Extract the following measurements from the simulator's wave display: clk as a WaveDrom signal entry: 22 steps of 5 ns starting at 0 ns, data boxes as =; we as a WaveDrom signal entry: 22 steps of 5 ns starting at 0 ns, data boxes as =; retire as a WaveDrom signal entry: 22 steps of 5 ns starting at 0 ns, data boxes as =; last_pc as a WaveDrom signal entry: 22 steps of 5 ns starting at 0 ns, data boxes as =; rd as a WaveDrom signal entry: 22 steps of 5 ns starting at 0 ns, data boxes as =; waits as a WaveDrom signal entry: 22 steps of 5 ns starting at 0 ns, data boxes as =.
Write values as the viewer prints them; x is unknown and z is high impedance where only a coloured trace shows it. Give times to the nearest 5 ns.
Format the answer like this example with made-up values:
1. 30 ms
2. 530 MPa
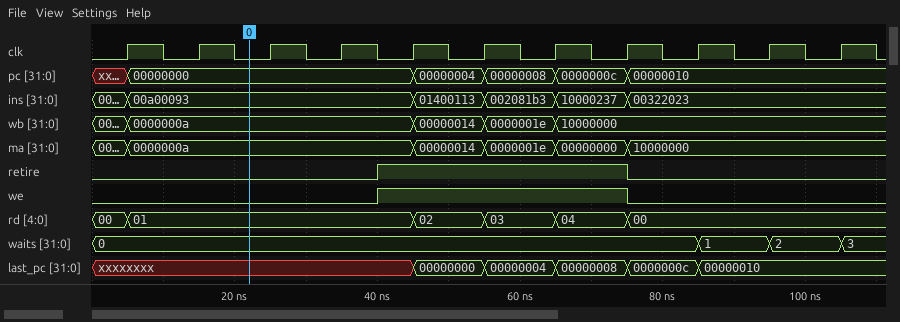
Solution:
1. {name: 'clk', wave: '0101010101010101010101'}
2. {name: 'we', wave: '0.......1......0......'}
3. {name: 'retire', wave: '0.......1......0......'}
4. {name: 'last_pc', wave: 'x........=.=.=.=.=....', data: '00000000 00000004 00000008 0000000c 00000010'}
5. {name: 'rd', wave: '==.......=.=.=.=......', data: '00 01 02 03 04 00'}
6. {name: 'waits', wave: '=................=.=.=', data: '0 1 2 3'}
